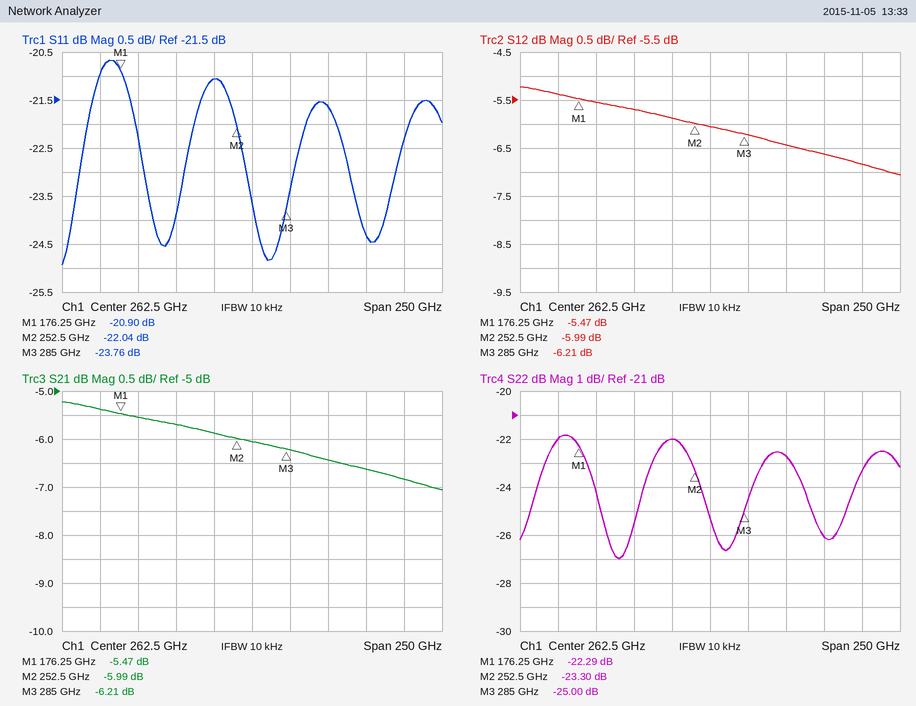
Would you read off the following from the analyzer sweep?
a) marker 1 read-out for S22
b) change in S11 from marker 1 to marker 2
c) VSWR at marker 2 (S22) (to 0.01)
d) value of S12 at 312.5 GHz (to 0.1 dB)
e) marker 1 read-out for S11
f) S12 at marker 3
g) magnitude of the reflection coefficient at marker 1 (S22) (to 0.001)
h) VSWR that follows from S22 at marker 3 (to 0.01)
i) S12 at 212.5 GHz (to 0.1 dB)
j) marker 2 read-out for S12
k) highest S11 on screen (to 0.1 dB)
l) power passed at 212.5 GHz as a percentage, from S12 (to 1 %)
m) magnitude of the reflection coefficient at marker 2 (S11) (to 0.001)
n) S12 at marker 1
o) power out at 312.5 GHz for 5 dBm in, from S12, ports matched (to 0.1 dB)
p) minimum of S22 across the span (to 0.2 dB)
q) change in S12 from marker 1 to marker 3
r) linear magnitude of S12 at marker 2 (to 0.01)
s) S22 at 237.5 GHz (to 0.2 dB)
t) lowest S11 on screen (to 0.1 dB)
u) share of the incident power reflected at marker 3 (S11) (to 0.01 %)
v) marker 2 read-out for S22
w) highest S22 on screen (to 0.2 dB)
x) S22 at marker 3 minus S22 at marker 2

-22.29 dB
-1.14 dB
1.15
-6.4 dB
-20.90 dB
-6.21 dB
0.077
1.12
-5.7 dB
-5.99 dB
-20.7 dB
27 %
0.079
-5.47 dB
-1.4 dBm
-27.0 dB
-0.74 dB
0.50
-22.0 dB
-24.9 dB
0.42 %
-23.30 dB
-21.8 dB
-1.70 dB
